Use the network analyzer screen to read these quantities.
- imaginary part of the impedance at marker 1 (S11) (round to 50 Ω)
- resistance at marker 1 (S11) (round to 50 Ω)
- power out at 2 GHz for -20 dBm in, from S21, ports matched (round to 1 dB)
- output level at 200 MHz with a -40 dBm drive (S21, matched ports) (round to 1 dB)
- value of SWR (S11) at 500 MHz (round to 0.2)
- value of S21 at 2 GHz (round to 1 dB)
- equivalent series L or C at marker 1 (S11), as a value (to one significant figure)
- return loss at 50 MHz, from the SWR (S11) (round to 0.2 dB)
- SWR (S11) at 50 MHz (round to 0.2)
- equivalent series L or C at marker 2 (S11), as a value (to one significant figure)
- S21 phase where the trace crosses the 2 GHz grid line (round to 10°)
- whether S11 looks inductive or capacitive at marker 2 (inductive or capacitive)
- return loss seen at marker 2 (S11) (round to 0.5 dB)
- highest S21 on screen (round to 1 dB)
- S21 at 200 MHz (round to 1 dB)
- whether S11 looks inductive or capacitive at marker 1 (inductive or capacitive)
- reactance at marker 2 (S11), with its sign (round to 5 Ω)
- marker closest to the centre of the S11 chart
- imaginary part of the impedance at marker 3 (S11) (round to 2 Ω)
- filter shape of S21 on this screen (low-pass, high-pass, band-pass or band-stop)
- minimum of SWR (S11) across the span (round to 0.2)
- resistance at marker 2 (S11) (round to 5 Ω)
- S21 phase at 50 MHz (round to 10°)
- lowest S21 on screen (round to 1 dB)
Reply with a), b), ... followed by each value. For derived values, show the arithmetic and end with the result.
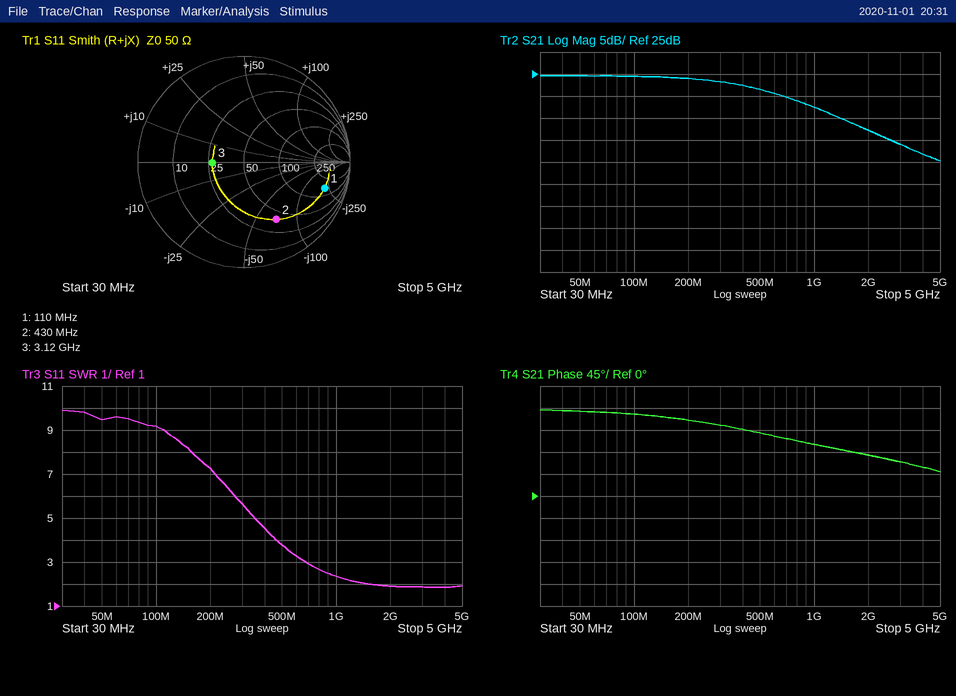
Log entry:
a) -200 Ω
b) 150 Ω
c) -20 dBm + (12 dB) = -8 dBm
d) -40 dBm + (24 dB) = -16 dBm
e) 3.8
f) 12 dB
g) C = 1/(2π × 110 MHz × 200 Ω) ≈ 7 pF
h) −20 log10((9.4 − 1)/(9.4 + 1)) ≈ 1.86 dB, so 1.8 dB to the nearest 0.2 dB
i) 9.4
j) C = 1/(2π × 430 MHz × 70 Ω) ≈ 5 pF
k) 80°
l) capacitive
m) 4.0 dB
n) 25 dB
o) 24 dB
p) capacitive
q) -70 Ω
r) marker 3
s) 0 Ω
t) low-pass
u) 1.8
v) 40 Ω
w) 170°
x) 5 dB
